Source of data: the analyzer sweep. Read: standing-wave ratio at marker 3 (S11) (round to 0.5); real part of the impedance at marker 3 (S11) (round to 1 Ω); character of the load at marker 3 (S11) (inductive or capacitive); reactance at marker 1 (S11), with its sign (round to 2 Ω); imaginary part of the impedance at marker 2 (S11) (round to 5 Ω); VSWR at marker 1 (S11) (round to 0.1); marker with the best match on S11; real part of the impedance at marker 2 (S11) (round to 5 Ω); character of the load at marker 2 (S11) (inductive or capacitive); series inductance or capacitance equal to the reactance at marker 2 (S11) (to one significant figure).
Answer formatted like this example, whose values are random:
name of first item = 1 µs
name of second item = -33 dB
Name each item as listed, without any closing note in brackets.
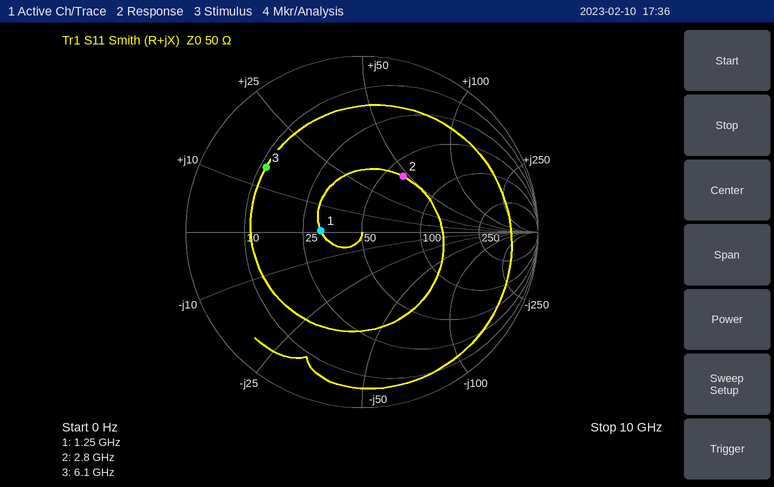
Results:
standing-wave ratio at marker 3 (S11) = 5.0
real part of the impedance at marker 3 (S11) = 11 Ω
character of the load at marker 3 (S11) = inductive
reactance at marker 1 (S11), with its sign = 0 Ω
imaginary part of the impedance at marker 2 (S11) = +45 Ω
VSWR at marker 1 (S11) = 1.6
marker with the best match on S11 = marker 1
real part of the impedance at marker 2 (S11) = 60 Ω
character of the load at marker 2 (S11) = inductive
series inductance or capacitance equal to the reactance at marker 2 (S11) = 3 nH
